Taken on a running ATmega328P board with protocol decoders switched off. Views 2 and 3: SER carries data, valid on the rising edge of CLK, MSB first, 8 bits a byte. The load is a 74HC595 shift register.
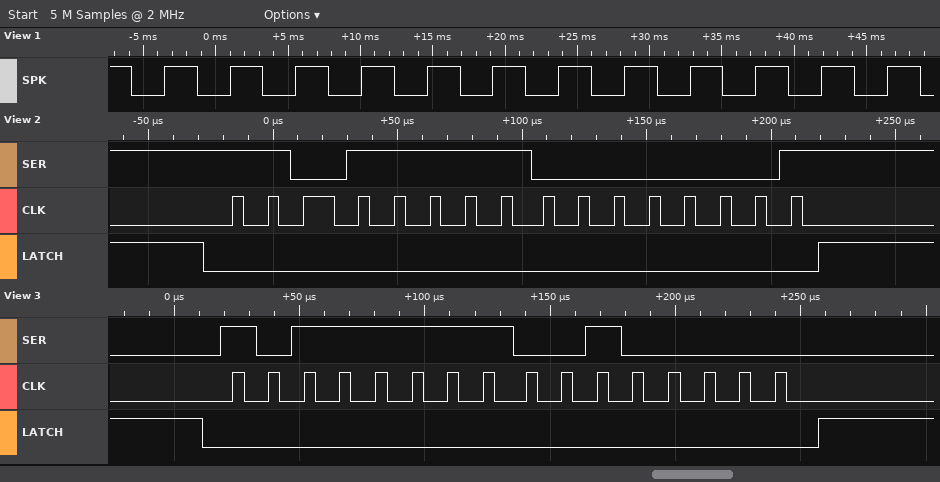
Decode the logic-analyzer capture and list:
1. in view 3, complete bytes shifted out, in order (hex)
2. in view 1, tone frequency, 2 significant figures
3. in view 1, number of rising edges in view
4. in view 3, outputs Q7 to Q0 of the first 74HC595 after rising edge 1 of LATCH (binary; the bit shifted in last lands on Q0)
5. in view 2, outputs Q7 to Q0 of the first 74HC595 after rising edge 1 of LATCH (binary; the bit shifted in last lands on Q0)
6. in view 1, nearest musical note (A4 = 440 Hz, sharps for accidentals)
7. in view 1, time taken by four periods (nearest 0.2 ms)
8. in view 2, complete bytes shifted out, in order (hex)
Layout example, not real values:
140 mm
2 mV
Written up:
BF 20
220 Hz
12
00100000
00000001
A3
18.2 ms
DF 01
